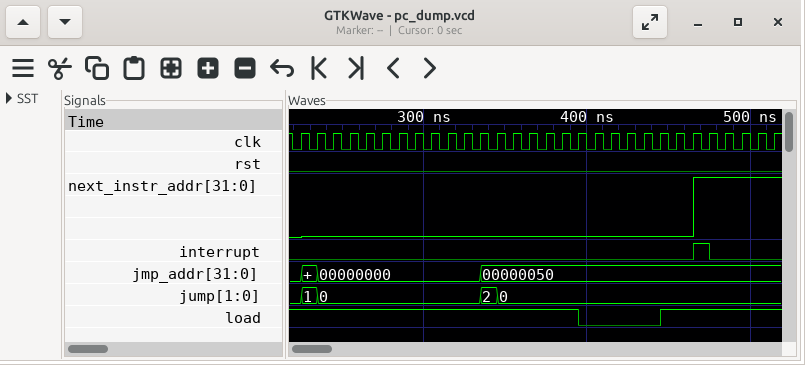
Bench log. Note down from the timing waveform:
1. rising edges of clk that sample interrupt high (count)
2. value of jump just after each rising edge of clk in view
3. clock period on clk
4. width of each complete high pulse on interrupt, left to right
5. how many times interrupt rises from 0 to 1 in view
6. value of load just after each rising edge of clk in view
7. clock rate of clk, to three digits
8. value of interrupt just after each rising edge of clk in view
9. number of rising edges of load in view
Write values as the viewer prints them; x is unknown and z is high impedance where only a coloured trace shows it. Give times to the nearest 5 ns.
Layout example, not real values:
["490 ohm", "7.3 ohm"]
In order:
["1", "1, 0, 0, 0, 0, 0, 0, 0, 0, 0, 0, 2, 0, 0, 0, 0, 0, 0, 0, 0, 0, 0, 0, 0, 0, 0, 0, 0, 0, 0", "10 ns", "10 ns", "1", "1 1 1 1 1 1 1 1 1 1 1 1 1 1 1 1 1 0 0 0 0 0 1 1 1 1 1 1 1 1", "100 MHz", "0 0 0 0 0 0 0 0 0 0 0 0 0 0 0 0 0 0 0 0 0 0 0 0 1 0 0 0 0 0", "1"]
